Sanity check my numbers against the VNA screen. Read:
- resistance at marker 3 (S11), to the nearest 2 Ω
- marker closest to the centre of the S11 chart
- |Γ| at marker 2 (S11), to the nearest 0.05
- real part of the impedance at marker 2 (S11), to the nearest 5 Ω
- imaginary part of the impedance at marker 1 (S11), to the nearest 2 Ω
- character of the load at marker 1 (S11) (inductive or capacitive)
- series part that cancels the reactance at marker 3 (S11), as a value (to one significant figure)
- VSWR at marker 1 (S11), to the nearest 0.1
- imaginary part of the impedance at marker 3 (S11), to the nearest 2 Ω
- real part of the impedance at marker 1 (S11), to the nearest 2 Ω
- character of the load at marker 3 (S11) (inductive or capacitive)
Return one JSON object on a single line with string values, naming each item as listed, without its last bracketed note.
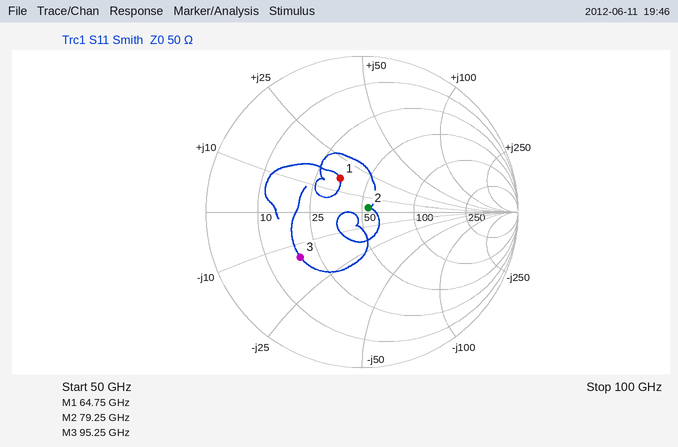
{"resistance at marker 3 (S11), to the nearest 2 Ω": "18 Ω", "marker closest to the centre of the S11 chart": "marker 2", "|Γ| at marker 2 (S11), to the nearest 0.05": "0.05", "real part of the impedance at marker 2 (S11), to the nearest 5 Ω": "55 Ω", "imaginary part of the impedance at marker 1 (S11), to the nearest 2 Ω": "+16 Ω", "character of the load at marker 1 (S11)": "inductive", "series part that cancels the reactance at marker 3 (S11), as a value": "20 pH", "VSWR at marker 1 (S11), to the nearest 0.1": "1.7", "imaginary part of the impedance at marker 3 (S11), to the nearest 2 Ω": "-14 Ω", "real part of the impedance at marker 1 (S11), to the nearest 2 Ω": "34 Ω", "character of the load at marker 3 (S11)": "capacitive"}
